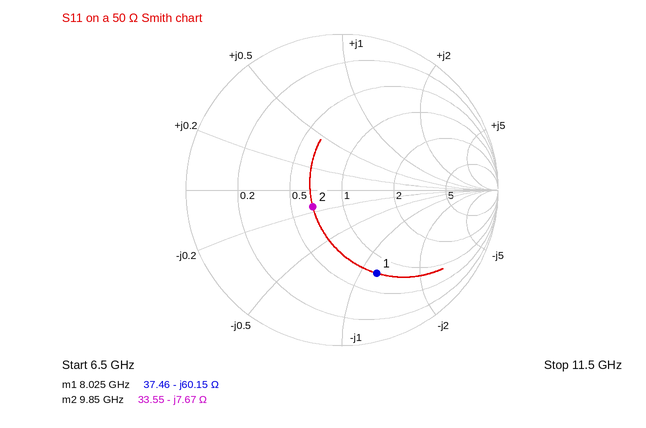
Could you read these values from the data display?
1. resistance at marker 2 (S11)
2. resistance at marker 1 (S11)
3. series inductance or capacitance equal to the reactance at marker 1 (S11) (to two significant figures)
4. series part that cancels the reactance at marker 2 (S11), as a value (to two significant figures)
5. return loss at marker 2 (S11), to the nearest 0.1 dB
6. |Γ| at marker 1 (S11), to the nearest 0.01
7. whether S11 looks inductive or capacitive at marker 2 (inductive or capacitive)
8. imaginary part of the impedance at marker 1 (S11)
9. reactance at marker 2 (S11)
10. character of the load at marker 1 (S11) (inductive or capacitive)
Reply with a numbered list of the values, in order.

1. 33.55 Ω
2. 37.46 Ω
3. 330 fF
4. 120 pH
5. 13.3 dB
6. 0.58
7. capacitive
8. -60.15 Ω
9. -7.67 Ω
10. capacitive
